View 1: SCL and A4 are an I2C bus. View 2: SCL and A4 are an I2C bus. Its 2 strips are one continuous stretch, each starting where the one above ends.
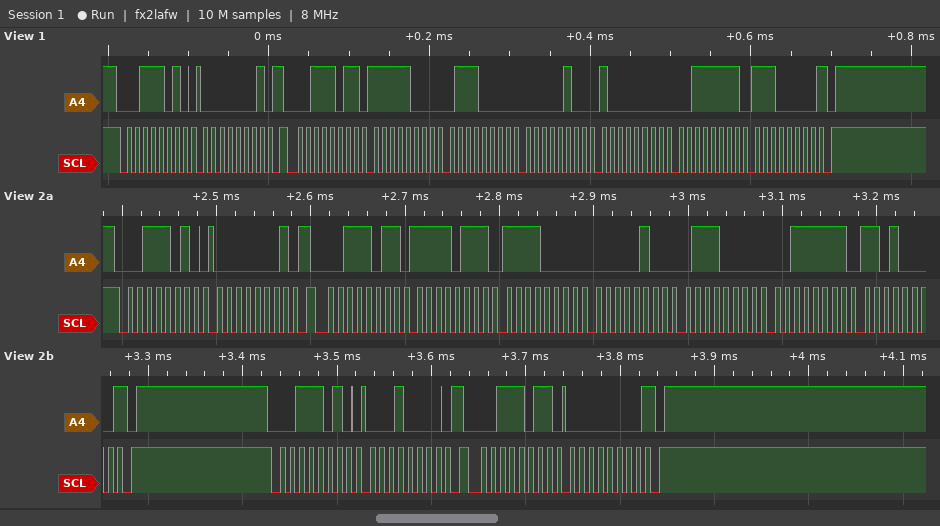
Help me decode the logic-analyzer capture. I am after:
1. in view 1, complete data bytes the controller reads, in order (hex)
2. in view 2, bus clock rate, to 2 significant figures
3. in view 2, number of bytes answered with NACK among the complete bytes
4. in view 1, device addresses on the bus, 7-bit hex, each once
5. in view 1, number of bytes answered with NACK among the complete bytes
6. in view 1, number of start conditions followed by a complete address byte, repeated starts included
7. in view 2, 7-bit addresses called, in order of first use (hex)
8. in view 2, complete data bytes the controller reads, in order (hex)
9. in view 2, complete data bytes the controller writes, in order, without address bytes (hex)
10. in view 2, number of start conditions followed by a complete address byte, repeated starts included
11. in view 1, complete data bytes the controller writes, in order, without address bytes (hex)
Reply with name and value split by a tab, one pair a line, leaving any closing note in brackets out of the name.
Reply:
in view 1, complete data bytes the controller reads, in order	F8 70 04 80 3F E0
in view 2, bus clock rate, to 2 significant figures	100 kHz
in view 2, number of bytes answered with NACK among the complete bytes	2
in view 1, device addresses on the bus, 7-bit hex, each once	0x1D
in view 1, number of bytes answered with NACK among the complete bytes	1
in view 1, number of start conditions followed by a complete address byte, repeated starts included	2
in view 2, 7-bit addresses called, in order of first use	0x1D
in view 2, complete data bytes the controller reads, in order	F7 F0 04 70 3F D0 00
in view 2, complete data bytes the controller writes, in order, without address bytes	01 10
in view 2, number of start conditions followed by a complete address byte, repeated starts included	4
in view 1, complete data bytes the controller writes, in order, without address bytes	01
